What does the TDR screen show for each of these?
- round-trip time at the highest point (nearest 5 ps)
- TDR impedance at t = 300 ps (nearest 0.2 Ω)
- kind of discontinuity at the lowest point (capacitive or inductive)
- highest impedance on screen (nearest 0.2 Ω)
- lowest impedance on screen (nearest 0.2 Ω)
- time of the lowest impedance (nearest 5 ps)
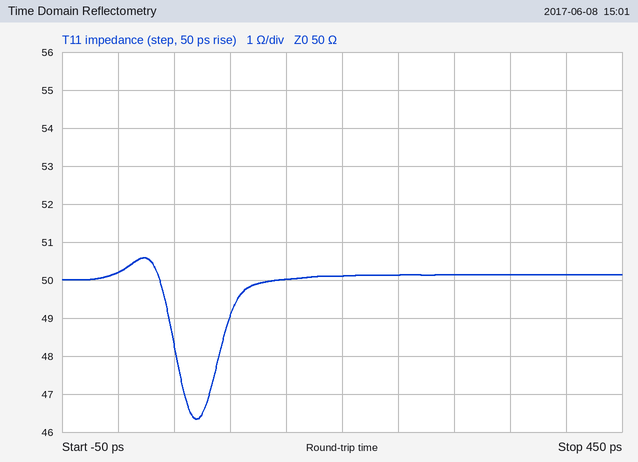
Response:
25 ps
50.2 Ω
capacitive
50.6 Ω
46.4 Ω
70 ps
